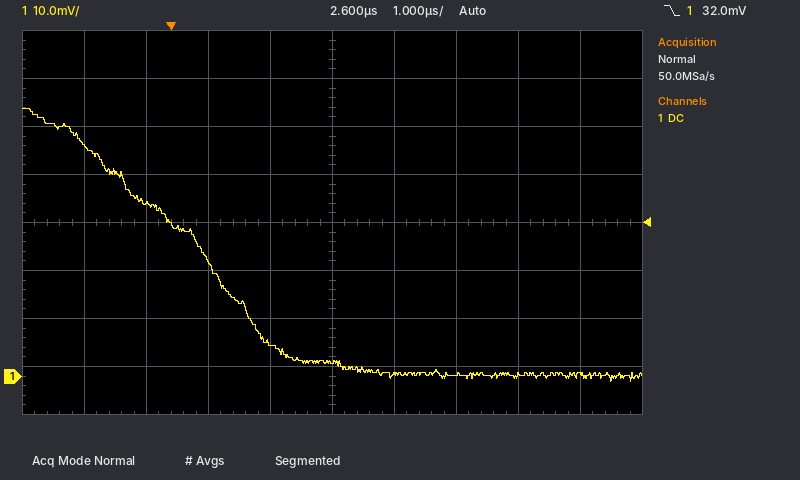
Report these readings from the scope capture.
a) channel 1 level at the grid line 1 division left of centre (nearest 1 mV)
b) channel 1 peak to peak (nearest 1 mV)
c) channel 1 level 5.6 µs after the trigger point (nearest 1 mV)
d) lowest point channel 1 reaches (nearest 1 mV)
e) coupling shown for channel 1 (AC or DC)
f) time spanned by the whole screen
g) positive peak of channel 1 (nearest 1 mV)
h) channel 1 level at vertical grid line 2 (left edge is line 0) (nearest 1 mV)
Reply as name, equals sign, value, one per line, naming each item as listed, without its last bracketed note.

channel 1 level at the grid line 1 division left of centre = 7 mV
channel 1 peak to peak = 57 mV
channel 1 level 5.6 µs after the trigger point = 0 mV
lowest point channel 1 reaches = -1 mV
coupling shown for channel 1 = DC
time spanned by the whole screen = 10 µs
positive peak of channel 1 = 56 mV
channel 1 level at vertical grid line 2 (left edge is line 0) = 36 mV
